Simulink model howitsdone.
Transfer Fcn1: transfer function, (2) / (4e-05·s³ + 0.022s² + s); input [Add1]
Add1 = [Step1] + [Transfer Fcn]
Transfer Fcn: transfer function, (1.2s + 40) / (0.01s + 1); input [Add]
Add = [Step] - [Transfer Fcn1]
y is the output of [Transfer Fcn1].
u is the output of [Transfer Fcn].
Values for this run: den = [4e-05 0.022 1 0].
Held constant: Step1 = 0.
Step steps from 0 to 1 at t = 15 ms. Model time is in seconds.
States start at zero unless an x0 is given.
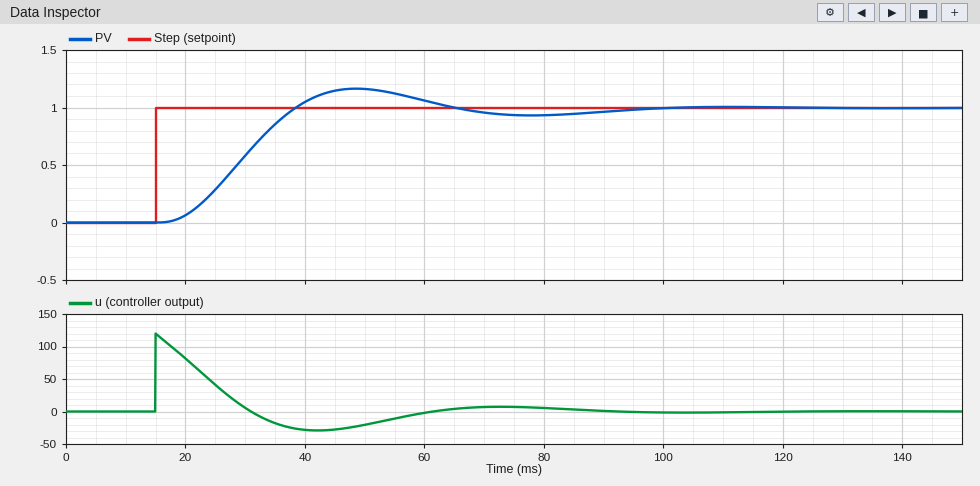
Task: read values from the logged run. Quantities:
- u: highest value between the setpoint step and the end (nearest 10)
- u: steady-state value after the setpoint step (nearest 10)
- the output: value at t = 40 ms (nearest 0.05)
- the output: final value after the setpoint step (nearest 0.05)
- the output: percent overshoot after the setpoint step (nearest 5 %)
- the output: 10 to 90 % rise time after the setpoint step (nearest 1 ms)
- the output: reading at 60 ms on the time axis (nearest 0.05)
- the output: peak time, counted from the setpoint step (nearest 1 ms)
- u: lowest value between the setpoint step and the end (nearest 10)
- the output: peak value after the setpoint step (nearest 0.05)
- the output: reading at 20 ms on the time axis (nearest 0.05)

120
0
1.05
1.00
15 %
15 ms
1.05
34 ms
-30
1.15
0.05
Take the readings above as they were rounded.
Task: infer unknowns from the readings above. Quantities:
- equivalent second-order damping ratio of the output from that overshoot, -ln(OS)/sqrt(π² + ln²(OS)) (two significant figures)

0.52
